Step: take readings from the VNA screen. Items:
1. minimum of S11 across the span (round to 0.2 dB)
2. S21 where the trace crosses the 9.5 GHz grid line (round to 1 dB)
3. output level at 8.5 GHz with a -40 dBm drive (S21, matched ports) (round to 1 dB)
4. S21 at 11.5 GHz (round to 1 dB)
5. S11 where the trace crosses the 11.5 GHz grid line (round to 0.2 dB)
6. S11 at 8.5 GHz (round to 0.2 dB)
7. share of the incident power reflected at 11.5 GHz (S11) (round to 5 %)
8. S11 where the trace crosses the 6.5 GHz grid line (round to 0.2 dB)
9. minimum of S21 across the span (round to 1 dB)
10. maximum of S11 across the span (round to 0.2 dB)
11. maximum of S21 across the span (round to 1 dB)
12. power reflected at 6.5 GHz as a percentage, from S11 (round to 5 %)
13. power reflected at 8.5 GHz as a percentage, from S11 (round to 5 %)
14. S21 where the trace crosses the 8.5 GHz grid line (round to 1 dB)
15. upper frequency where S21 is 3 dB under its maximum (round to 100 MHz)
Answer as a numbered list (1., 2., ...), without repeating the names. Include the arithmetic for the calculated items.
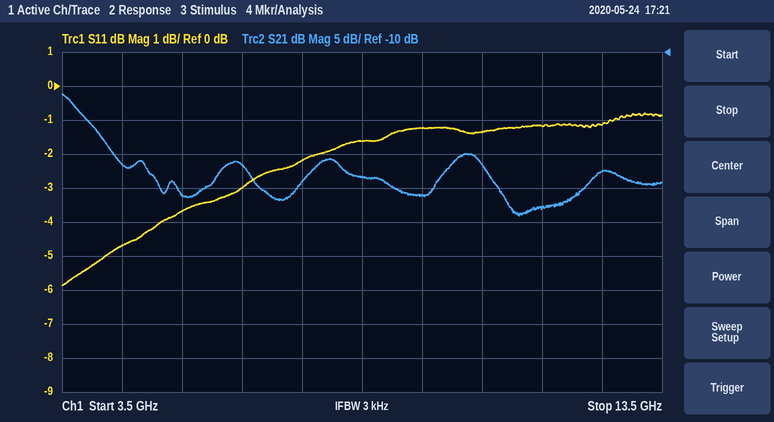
1. -5.8 dB
2. -31 dB
3. -40 dBm + (-28 dB) = -68 dBm
4. -33 dB
5. -1.2 dB
6. -1.6 dB
7. 10^(-1.2/10) ≈ 75.9 %, so 75 % to the nearest 5 %
8. -3.0 dB
9. -34 dB
10. -0.8 dB
11. -16 dB
12. 10^(-3/10) ≈ 50 %
13. 10^(-1.6/10) ≈ 69.2 %, so 70 % to the nearest 5 %
14. -28 dB
15. 3.8 GHz
